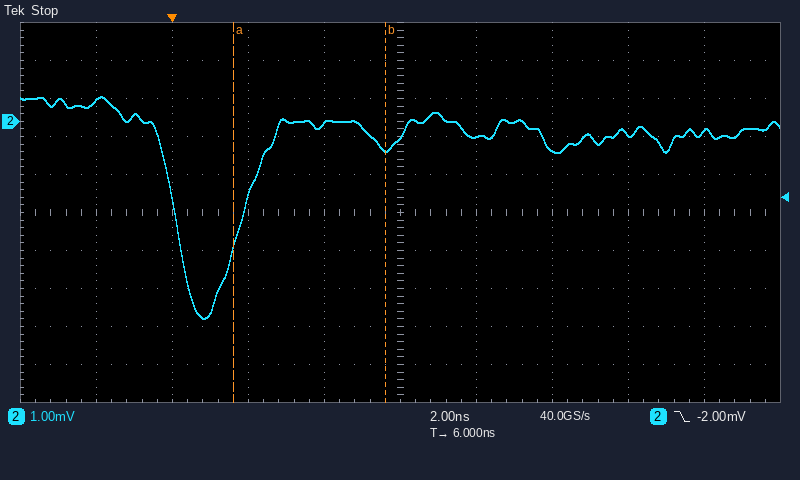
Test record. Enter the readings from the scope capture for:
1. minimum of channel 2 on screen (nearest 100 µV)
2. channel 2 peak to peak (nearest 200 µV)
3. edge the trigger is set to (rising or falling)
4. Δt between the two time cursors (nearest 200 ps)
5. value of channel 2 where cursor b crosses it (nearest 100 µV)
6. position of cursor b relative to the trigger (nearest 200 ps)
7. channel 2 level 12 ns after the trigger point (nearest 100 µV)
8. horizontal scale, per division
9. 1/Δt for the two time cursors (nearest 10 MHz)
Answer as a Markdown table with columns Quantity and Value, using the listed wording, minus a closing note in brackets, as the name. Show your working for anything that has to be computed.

| Quantity | Value |
|---|---|
| minimum of channel 2 on screen | -5.2 mV |
| channel 2 peak to peak | 5.8 mV |
| edge the trigger is set to | falling |
| Δt between the two time cursors | 4.0 ns |
| value of channel 2 where cursor b crosses it | -800 µV |
| position of cursor b relative to the trigger | +5.6 ns |
| channel 2 level 12 ns after the trigger point | -300 µV |
| horizontal scale, per division | 2 ns |
| 1/Δt for the two time cursors | 1 / 4.0 ns ≈ 250 MHz |
